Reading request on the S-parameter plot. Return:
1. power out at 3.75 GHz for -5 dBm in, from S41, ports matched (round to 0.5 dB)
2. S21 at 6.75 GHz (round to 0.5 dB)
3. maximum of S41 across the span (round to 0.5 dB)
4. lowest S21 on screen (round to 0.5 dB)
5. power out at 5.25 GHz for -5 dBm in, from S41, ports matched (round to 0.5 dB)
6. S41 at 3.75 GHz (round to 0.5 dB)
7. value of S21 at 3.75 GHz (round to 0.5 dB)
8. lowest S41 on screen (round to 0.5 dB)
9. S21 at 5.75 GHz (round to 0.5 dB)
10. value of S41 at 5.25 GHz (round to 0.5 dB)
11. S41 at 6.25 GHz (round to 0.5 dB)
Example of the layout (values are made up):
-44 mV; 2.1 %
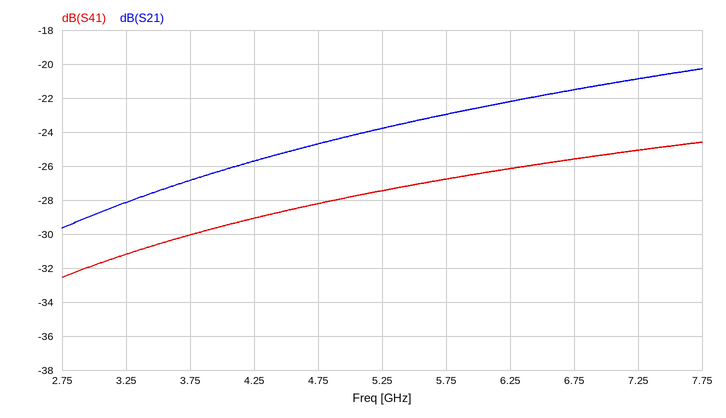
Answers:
-35.0 dBm; -21.5 dB; -24.5 dB; -29.5 dB; -32.5 dBm; -30.0 dB; -27.0 dB; -32.5 dB; -23.0 dB; -27.5 dB; -26.0 dB
